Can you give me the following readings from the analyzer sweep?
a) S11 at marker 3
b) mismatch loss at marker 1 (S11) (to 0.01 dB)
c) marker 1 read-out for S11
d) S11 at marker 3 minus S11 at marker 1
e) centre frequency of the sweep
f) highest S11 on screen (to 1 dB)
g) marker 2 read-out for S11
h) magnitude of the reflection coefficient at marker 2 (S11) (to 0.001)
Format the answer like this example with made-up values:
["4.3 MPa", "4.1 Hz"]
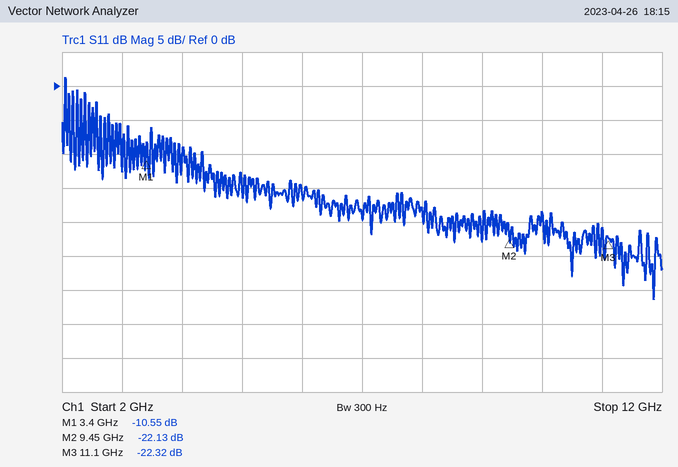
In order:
["-22.32 dB", "0.40 dB", "-10.55 dB", "-11.77 dB", "7 GHz", "1 dB", "-22.13 dB", "0.078"]
